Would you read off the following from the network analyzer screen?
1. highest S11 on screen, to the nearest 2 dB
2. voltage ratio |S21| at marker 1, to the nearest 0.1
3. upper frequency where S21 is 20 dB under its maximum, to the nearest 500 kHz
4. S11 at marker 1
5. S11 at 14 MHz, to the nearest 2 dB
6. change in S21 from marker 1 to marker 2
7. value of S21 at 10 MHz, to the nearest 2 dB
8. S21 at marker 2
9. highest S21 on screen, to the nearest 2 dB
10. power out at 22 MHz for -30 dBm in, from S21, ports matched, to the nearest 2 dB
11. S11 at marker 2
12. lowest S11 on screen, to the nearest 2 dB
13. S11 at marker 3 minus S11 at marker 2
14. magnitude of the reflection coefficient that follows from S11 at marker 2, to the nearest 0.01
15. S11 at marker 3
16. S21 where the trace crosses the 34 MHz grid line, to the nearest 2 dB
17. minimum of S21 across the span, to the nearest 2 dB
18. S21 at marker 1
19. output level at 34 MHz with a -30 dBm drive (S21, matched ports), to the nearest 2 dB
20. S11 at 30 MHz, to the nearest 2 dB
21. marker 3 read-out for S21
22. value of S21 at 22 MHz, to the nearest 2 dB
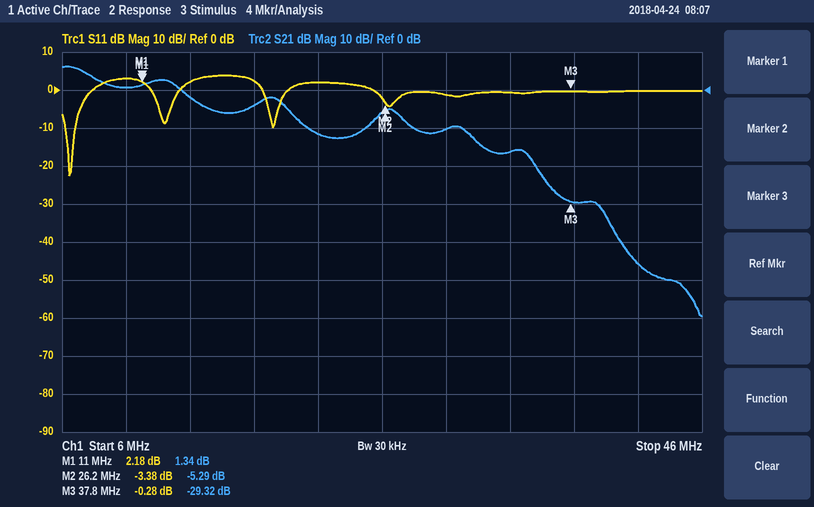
4 dB
1.2
32.0 MHz
2.18 dB
2 dB
-6.63 dB
0 dB
-5.29 dB
6 dB
-42 dBm
-3.38 dB
-22 dB
3.10 dB
0.68
-0.28 dB
-16 dB
-60 dB
1.34 dB
-46 dBm
-2 dB
-29.32 dB
-12 dB
